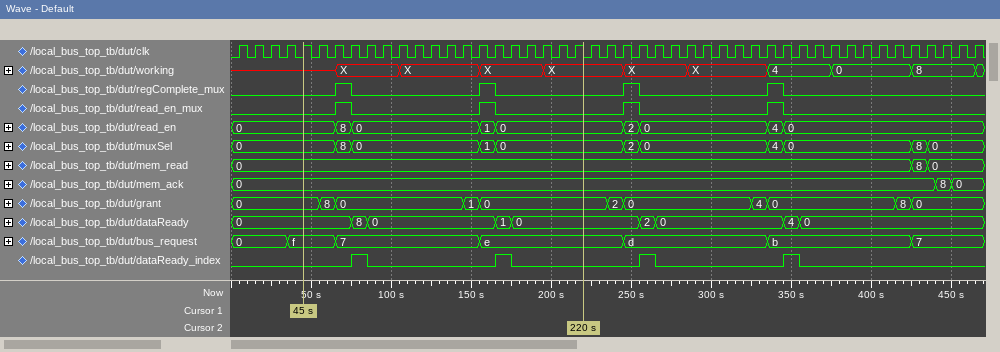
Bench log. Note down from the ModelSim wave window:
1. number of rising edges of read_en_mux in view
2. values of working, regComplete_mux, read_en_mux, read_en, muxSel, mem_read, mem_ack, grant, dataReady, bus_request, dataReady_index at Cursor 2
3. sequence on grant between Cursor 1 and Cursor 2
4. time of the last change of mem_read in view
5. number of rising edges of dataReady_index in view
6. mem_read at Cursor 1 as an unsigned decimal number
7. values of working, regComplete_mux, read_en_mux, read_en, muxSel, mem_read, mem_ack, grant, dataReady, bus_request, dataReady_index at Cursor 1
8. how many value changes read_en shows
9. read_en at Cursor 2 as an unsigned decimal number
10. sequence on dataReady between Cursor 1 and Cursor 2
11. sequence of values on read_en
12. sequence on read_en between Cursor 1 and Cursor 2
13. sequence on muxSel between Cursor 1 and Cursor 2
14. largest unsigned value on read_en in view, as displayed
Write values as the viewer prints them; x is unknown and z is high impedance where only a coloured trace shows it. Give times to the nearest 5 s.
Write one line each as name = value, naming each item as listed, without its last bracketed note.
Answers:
number of rising edges of read_en_mux in view = 4
values of working, regComplete_mux, read_en_mux, read_en, muxSel, mem_read, mem_ack, grant, dataReady, bus_request, dataReady_index at Cursor 2 = working=X, regComplete_mux=0, read_en_mux=0, read_en=0, muxSel=0, mem_read=0, mem_ack=0, grant=0, dataReady=0, bus_request=e, dataReady_index=0
sequence on grant between Cursor 1 and Cursor 2 = 0, 8, 0, 1, 0
time of the last change of mem_read in view = 435 s
number of rising edges of dataReady_index in view = 4
mem_read at Cursor 1 as an unsigned decimal number = 0
values of working, regComplete_mux, read_en_mux, read_en, muxSel, mem_read, mem_ack, grant, dataReady, bus_request, dataReady_index at Cursor 1 = working=x, regComplete_mux=0, read_en_mux=0, read_en=0, muxSel=0, mem_read=0, mem_ack=0, grant=0, dataReady=0, bus_request=f, dataReady_index=0
how many value changes read_en shows = 8
read_en at Cursor 2 as an unsigned decimal number = 0
sequence on dataReady between Cursor 1 and Cursor 2 = 0, 8, 0, 1, 0
sequence of values on read_en = 0, 8, 0, 1, 0, 2, 0, 4, 0
sequence on read_en between Cursor 1 and Cursor 2 = 0, 8, 0, 1, 0
sequence on muxSel between Cursor 1 and Cursor 2 = 0, 8, 0, 1, 0
largest unsigned value on read_en in view, as displayed = 8
